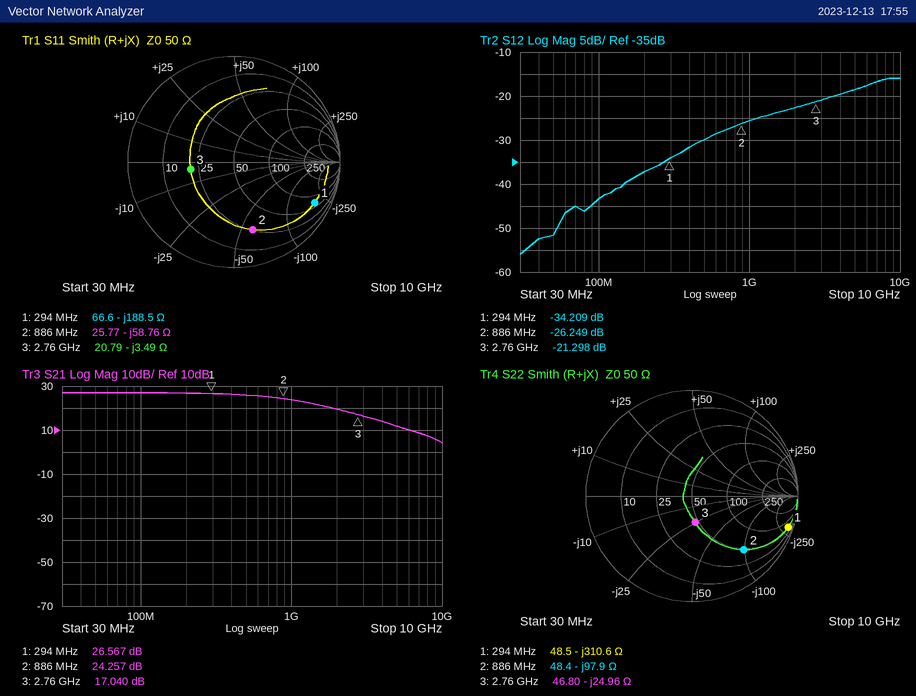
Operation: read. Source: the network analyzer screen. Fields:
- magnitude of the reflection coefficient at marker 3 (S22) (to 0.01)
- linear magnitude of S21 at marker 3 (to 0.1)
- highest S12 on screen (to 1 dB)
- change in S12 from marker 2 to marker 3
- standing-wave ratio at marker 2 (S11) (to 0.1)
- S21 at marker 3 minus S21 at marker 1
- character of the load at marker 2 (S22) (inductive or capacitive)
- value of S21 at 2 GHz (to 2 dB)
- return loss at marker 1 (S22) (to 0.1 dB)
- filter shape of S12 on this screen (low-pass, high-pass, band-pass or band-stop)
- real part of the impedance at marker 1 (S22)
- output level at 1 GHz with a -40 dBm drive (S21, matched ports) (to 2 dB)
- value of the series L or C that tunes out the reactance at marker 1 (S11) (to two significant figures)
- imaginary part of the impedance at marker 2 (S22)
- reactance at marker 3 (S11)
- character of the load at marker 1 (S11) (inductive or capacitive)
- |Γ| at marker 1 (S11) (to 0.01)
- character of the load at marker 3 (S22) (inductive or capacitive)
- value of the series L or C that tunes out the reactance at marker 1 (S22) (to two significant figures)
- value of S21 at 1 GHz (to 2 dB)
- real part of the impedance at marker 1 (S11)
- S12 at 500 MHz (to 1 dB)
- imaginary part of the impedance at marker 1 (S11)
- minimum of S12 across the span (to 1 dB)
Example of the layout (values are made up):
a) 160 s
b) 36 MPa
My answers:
a) 0.25
b) 7.1
c) -16 dB
d) 4.951 dB
e) 4.9
f) -9.527 dB
g) capacitive
h) 20 dB
i) 0.4 dB
j) high-pass
k) 48.5 Ω
l) -16 dBm
m) 100 nH
n) -97.9 Ω
o) -3.49 Ω
p) capacitive
q) 0.85
r) capacitive
s) 170 nH
t) 24 dB
u) 66.6 Ω
v) -30 dB
w) -188.5 Ω
x) -56 dB
